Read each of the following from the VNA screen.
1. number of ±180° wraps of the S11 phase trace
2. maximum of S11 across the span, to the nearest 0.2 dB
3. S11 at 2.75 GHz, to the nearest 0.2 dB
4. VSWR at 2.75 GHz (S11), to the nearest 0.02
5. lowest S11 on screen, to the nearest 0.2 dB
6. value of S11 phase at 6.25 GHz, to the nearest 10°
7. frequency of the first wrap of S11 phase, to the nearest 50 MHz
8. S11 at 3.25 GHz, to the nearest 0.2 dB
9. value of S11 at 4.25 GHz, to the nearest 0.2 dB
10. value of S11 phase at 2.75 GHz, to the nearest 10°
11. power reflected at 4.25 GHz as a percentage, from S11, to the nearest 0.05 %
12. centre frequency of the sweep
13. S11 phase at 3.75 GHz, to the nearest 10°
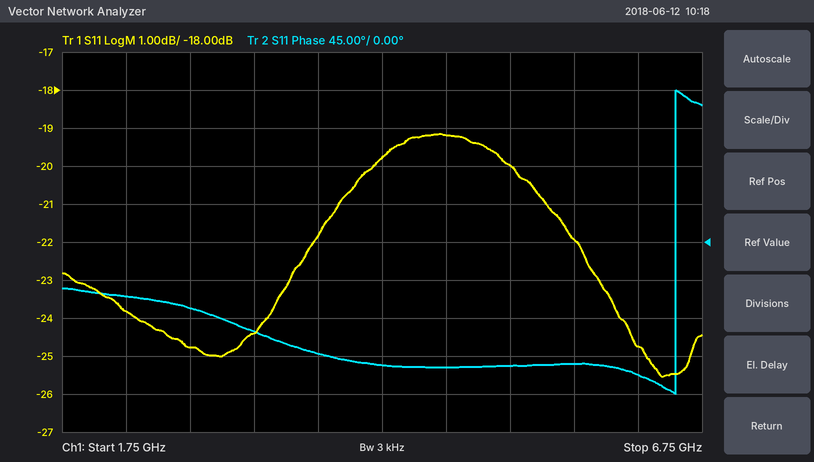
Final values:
1
-19.2 dB
-24.8 dB
1.12
-25.6 dB
-160°
6.55 GHz
-24.4 dB
-19.8 dB
-80°
1.05 %
4.25 GHz
-130°
